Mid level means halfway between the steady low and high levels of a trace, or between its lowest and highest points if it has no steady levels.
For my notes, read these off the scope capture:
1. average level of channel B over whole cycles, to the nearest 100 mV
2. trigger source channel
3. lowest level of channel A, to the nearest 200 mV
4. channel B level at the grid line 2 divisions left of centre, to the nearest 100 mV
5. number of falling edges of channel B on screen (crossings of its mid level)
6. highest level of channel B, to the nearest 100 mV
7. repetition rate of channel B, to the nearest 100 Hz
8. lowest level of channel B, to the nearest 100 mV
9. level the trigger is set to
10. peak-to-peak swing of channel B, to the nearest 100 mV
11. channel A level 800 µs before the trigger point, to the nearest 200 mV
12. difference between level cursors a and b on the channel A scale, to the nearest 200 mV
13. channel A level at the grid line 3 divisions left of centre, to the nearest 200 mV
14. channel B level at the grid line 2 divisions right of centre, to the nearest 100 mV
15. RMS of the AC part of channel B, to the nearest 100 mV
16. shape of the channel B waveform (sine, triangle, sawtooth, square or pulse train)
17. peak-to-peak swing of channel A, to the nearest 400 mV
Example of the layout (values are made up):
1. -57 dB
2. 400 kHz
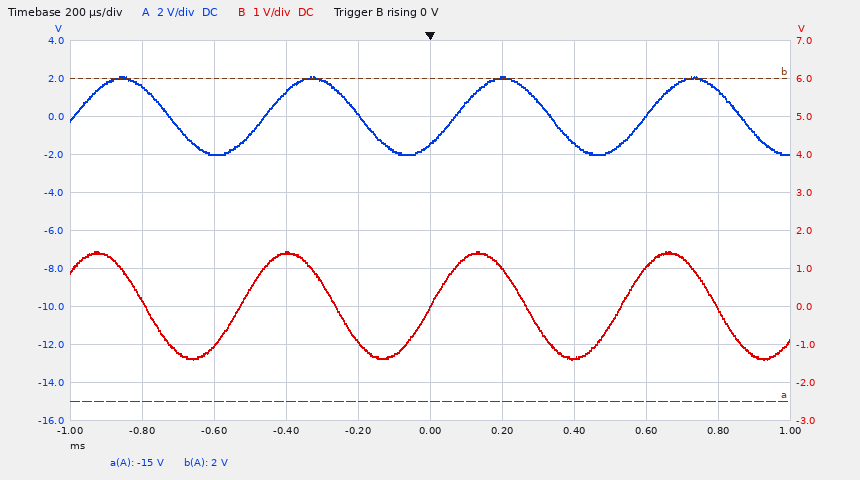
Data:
1. 0.0 V
2. channel B
3. -2.0 V
4. 1.4 V
5. 4
6. 1.4 V
7. 1.9 kHz
8. -1.4 V
9. 0 V
10. 2.8 V
11. 1.6 V
12. 17.0 V
13. -2.0 V
14. -1.4 V
15. 1.0 V
16. sine
17. 4.0 V
